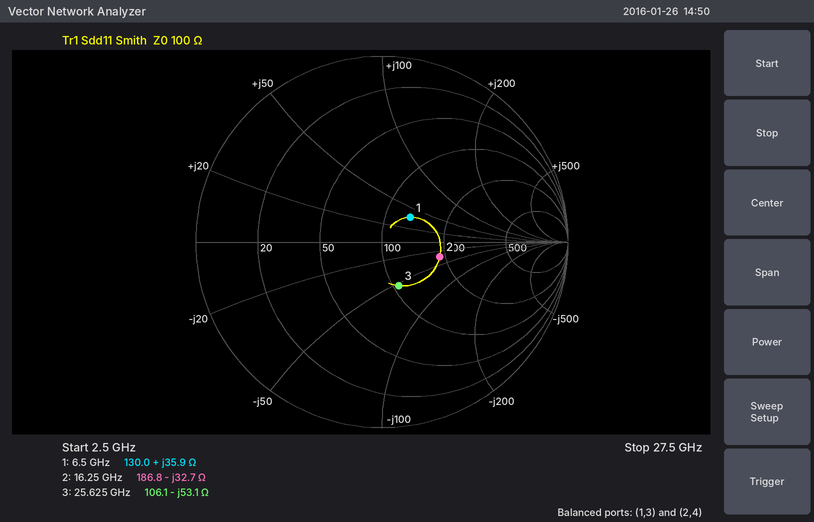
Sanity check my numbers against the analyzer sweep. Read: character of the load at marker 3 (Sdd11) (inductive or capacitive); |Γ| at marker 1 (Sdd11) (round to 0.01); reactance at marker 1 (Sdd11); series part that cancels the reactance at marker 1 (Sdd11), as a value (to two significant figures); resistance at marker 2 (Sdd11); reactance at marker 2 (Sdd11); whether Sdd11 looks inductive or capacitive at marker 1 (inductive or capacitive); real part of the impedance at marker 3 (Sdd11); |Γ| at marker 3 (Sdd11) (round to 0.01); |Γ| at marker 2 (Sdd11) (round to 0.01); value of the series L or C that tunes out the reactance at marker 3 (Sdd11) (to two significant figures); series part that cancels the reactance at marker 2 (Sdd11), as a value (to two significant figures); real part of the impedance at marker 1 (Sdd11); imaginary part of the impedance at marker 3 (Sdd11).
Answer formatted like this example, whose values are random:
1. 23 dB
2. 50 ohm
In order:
1. capacitive
2. 0.20
3. +35.9 Ω
4. 680 fF
5. 186.8 Ω
6. -32.7 Ω
7. inductive
8. 106.1 Ω
9. 0.25
10. 0.32
11. 330 pH
12. 320 pH
13. 130.0 Ω
14. -53.1 Ω
